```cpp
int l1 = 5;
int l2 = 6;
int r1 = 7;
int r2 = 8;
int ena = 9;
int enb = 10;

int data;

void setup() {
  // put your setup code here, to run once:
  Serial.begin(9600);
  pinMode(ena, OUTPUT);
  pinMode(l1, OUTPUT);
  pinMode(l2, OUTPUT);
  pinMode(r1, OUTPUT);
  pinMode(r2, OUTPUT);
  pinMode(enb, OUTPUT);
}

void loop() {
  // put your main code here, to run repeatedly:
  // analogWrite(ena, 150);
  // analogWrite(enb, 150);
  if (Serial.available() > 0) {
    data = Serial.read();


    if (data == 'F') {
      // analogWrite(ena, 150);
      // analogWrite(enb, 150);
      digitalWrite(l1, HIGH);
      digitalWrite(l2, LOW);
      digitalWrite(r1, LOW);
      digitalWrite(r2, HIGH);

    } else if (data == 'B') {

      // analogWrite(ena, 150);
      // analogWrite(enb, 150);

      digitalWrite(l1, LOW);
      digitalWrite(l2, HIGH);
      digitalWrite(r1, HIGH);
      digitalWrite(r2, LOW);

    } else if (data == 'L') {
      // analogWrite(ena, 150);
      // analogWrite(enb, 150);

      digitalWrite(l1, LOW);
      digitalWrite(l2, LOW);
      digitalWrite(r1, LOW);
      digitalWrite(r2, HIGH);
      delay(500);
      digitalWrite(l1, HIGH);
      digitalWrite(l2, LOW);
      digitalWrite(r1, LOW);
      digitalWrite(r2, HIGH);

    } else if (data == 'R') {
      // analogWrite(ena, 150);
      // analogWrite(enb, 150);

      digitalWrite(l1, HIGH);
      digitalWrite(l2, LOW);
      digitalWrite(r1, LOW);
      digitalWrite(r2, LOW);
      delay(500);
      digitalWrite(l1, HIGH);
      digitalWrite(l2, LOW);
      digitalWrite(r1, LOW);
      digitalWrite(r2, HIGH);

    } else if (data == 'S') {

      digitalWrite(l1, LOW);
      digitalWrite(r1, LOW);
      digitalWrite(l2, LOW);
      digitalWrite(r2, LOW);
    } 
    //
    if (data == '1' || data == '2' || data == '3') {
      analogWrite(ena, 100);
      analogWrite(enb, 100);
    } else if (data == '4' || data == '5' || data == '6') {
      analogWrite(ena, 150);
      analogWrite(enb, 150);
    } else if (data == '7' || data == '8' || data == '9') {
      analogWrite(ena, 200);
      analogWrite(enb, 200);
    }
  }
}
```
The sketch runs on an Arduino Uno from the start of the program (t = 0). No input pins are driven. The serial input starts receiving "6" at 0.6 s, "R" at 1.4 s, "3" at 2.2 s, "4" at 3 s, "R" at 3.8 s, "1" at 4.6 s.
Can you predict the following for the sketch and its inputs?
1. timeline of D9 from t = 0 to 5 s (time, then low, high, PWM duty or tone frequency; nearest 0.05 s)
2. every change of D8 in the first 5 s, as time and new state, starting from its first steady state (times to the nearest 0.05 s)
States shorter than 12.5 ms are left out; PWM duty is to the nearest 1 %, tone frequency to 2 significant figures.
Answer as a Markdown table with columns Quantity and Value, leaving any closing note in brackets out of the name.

| Quantity | Value |
|---|---|
| timeline of D9 from t = 0 to 5 s | 0 s low; 0.6 s PWM 59 %; 2.2 s PWM 39 %; 3 s PWM 59 %; 4.6 s PWM 39 % |
| every change of D8 in the first 5 s, as time and new state, starting from its first steady state | 0 s low; 1.9 s high; 3.8 s low; 4.3 s high |
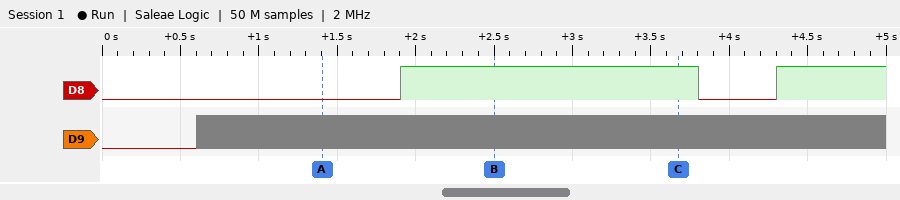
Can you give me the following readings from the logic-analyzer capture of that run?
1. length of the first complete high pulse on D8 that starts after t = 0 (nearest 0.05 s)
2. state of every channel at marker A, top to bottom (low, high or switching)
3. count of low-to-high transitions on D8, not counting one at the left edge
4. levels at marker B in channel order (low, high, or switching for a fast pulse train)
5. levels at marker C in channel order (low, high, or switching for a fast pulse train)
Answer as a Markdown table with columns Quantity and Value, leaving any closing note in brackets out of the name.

| Quantity | Value |
|---|---|
| length of the first complete high pulse on D8 that starts after t = 0 | 1.90 s |
| state of every channel at marker A, top to bottom | D8 low, D9 switching |
| count of low-to-high transitions on D8, not counting one at the left edge | 2 |
| levels at marker B in channel order | D8 high, D9 switching |
| levels at marker C in channel order | D8 high, D9 switching |
